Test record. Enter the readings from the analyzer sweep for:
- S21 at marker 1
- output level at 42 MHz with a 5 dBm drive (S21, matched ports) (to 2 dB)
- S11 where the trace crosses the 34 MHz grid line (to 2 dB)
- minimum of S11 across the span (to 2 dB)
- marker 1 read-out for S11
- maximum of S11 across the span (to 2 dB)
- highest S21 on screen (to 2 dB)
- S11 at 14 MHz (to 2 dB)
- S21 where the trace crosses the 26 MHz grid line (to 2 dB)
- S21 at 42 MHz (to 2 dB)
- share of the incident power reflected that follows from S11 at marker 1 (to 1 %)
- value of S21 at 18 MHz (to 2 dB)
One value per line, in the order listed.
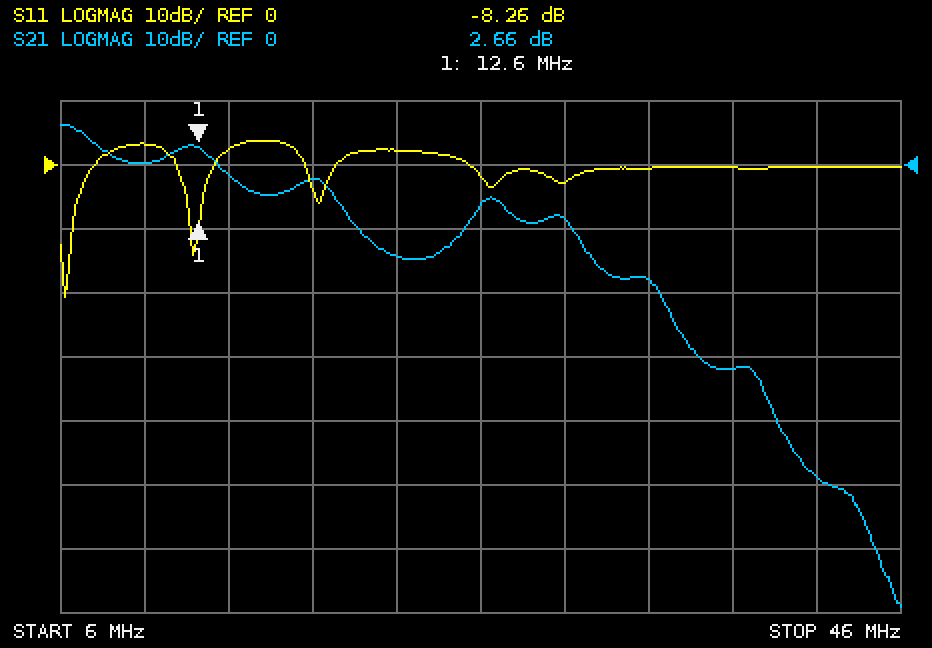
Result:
2.66 dB
-44 dBm
0 dB
-20 dB
-8.26 dB
4 dB
6 dB
2 dB
-6 dB
-48 dB
15 %
-2 dB
